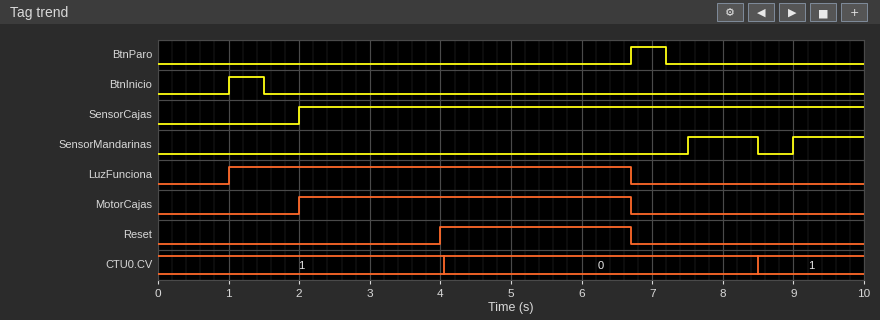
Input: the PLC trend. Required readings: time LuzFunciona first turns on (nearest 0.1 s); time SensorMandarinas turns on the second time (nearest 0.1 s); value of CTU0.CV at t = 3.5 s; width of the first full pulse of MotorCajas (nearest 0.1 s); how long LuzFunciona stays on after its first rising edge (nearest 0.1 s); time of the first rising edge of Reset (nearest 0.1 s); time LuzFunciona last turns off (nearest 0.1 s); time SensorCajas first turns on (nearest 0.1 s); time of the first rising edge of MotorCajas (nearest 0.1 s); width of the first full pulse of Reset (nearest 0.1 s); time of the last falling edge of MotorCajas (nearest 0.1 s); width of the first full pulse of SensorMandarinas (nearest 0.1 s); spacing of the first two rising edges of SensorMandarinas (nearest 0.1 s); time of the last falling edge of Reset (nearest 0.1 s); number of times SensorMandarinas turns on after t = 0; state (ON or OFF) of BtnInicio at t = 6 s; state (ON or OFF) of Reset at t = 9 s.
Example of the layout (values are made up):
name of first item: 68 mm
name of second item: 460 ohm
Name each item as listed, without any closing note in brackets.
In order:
time LuzFunciona first turns on: 1.0 s
time SensorMandarinas turns on the second time: 9.0 s
value of CTU0.CV at t = 3.5 s: 1
width of the first full pulse of MotorCajas: 4.7 s
how long LuzFunciona stays on after its first rising edge: 5.7 s
time of the first rising edge of Reset: 4.0 s
time LuzFunciona last turns off: 6.7 s
time SensorCajas first turns on: 2.0 s
time of the first rising edge of MotorCajas: 2.0 s
width of the first full pulse of Reset: 2.7 s
time of the last falling edge of MotorCajas: 6.7 s
width of the first full pulse of SensorMandarinas: 1.0 s
spacing of the first two rising edges of SensorMandarinas: 1.5 s
time of the last falling edge of Reset: 6.7 s
number of times SensorMandarinas turns on after t = 0: 2
state (ON or OFF) of BtnInicio at t = 6 s: OFF
state (ON or OFF) of Reset at t = 9 s: OFF
